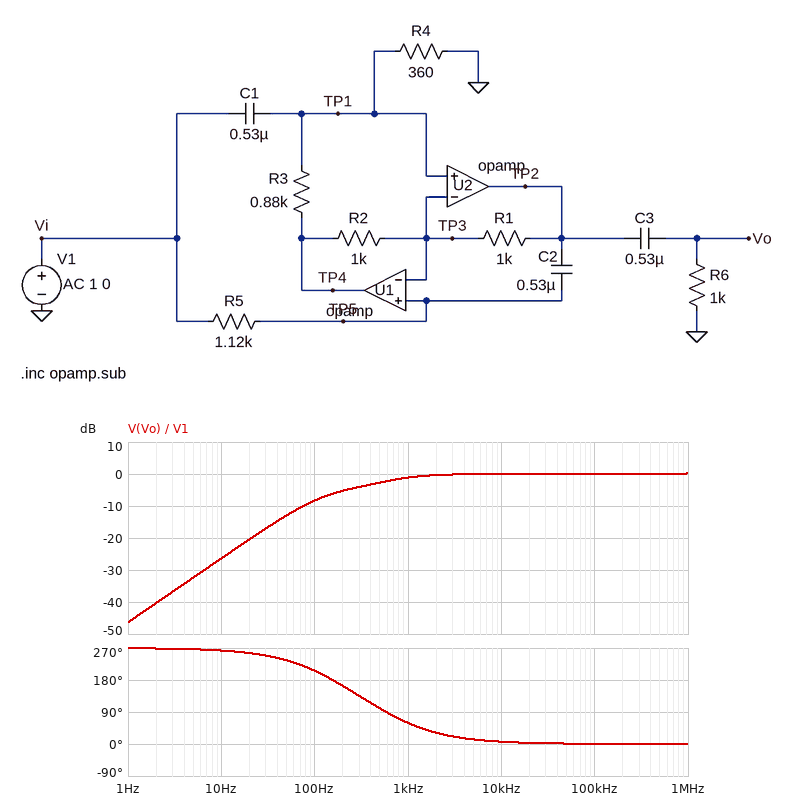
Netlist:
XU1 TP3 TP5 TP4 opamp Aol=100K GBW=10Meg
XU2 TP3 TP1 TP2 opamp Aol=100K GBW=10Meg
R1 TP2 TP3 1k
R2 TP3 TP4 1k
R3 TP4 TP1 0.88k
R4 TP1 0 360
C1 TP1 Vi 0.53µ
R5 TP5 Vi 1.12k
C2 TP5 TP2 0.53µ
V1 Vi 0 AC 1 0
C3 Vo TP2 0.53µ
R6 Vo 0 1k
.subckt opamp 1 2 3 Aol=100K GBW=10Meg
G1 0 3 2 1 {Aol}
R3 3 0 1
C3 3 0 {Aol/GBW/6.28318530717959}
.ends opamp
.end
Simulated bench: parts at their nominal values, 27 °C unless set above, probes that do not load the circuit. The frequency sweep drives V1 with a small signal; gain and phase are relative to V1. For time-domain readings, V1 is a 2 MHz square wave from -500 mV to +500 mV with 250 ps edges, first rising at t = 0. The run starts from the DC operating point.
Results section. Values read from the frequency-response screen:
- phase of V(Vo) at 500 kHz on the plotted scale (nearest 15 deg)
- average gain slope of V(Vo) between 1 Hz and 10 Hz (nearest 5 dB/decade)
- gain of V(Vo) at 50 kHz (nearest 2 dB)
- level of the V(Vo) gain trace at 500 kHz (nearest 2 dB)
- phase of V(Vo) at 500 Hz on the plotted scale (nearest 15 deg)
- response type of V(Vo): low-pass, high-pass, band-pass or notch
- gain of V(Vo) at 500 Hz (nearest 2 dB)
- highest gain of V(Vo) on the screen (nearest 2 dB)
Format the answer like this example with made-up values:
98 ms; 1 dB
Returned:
0 deg; 20 dB/decade; 0 dB; 0 dB; 105 deg; high-pass; -2 dB; 0 dB
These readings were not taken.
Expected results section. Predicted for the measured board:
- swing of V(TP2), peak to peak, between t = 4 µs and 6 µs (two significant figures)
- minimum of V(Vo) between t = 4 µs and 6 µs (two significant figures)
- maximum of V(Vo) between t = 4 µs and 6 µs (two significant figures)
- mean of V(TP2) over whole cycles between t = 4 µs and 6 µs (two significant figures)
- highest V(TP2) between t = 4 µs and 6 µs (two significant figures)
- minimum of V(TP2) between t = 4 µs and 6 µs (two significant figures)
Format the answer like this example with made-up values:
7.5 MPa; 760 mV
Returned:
1.4 V; -230 mV; 1.2 V; 1.2 V; 1.9 V; 500 mV
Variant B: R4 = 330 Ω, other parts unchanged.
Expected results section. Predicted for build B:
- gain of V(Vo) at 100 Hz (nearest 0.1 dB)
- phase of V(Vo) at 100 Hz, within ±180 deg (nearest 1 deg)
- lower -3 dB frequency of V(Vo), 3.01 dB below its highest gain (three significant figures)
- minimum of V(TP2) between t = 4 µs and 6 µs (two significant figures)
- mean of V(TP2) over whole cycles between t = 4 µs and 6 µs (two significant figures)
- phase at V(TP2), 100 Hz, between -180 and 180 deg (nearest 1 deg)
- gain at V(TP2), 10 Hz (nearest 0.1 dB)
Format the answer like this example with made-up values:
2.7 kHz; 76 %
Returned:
-7.5 dB; -157 deg; 1.27 kHz; 610 mV; 1.3 V; 132 deg; 4.4 dB
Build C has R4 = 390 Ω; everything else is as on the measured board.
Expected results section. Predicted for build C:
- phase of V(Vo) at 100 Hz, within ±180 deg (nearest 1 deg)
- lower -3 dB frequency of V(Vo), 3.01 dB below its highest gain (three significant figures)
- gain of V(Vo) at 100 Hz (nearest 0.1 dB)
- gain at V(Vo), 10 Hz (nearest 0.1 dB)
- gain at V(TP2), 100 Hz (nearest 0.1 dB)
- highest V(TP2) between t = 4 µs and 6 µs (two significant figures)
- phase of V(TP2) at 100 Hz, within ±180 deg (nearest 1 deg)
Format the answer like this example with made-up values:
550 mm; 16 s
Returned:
-152 deg; 1.02 kHz; -9.1 dB; -27.6 dB; 0.9 dB; 1.8 V; 137 deg
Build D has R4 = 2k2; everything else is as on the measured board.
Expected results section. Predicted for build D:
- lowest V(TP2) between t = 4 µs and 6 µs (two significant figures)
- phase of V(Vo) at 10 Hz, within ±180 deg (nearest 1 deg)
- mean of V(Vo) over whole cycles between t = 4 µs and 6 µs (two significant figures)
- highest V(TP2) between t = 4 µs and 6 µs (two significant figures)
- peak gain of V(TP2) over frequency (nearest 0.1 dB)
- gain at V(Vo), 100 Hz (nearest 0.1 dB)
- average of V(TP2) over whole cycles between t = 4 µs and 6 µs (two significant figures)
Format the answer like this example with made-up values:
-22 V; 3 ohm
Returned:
-510 mV; 87 deg; 490 mV; 910 mV; 2.1 dB; -15.3 dB; 200 mV
